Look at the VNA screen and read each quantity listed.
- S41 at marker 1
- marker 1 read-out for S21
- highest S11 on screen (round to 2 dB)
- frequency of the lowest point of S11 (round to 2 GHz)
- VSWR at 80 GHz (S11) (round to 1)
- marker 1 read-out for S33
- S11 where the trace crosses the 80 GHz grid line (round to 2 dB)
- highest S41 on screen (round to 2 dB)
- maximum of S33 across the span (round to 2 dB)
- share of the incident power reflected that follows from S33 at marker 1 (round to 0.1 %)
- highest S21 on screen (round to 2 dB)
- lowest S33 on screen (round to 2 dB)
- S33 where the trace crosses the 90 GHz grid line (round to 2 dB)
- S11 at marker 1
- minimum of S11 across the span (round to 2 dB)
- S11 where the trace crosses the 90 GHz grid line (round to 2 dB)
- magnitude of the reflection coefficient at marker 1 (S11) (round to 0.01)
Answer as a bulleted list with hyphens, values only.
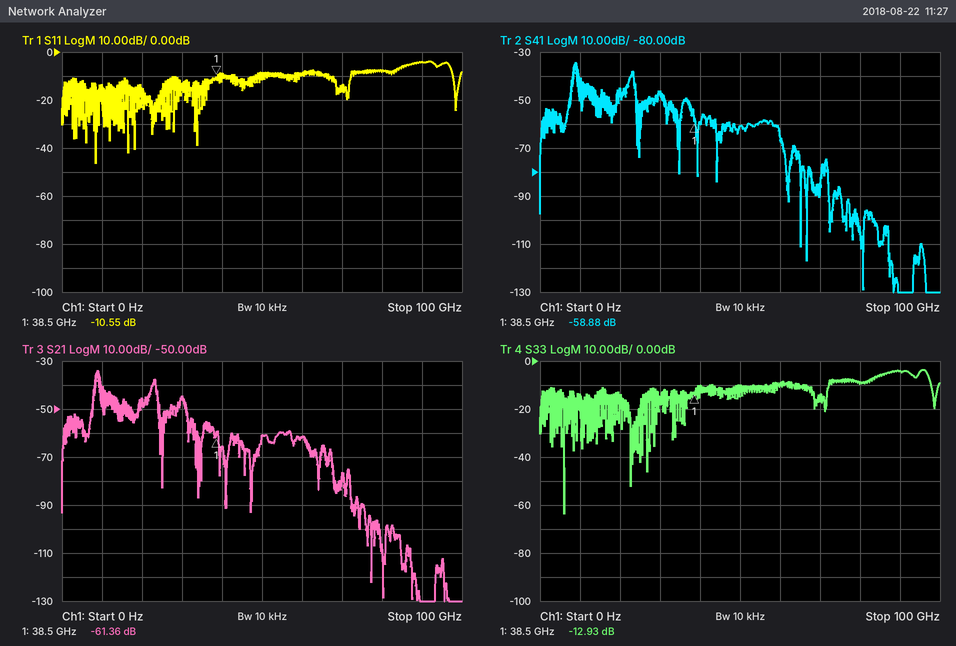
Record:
- -58.88 dB
- -61.36 dB
- -4 dB
- 8 GHz
- 2
- -12.93 dB
- -8 dB
- -34 dB
- -4 dB
- 5.1 %
- -34 dB
- -64 dB
- -4 dB
- -10.55 dB
- -46 dB
- -4 dB
- 0.30
